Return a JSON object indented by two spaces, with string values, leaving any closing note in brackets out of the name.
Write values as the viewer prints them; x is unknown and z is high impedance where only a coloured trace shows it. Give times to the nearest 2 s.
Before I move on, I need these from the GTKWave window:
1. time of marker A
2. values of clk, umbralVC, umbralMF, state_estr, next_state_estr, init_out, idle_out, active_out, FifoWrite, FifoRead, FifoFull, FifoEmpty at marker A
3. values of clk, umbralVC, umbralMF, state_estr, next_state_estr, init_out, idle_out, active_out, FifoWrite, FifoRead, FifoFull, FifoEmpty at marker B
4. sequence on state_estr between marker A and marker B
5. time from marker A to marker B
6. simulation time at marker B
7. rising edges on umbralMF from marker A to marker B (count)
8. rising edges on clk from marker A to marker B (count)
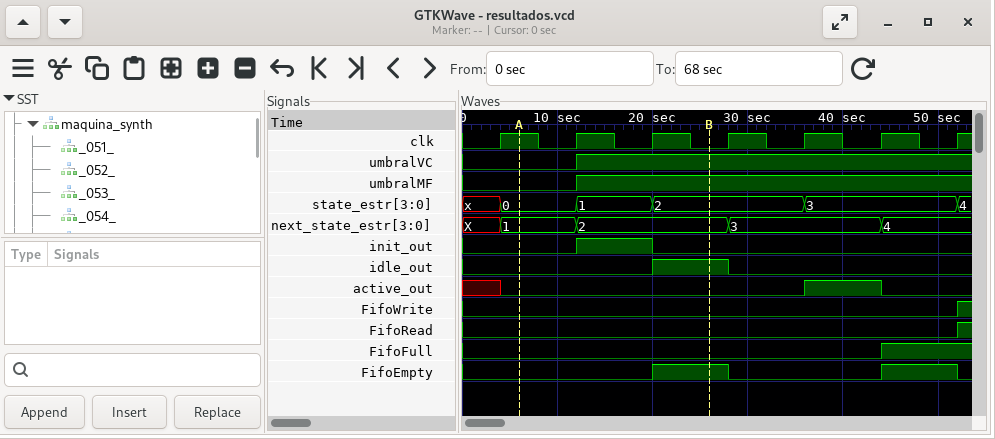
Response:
{
  "time of marker A": "6 s",
  "values of clk, umbralVC, umbralMF, state_estr, next_state_estr, init_out, idle_out, active_out, FifoWrite, FifoRead, FifoFull, FifoEmpty at marker A": "clk=1, umbralVC=0, umbralMF=0, state_estr=0, next_state_estr=1, init_out=0, idle_out=0, active_out=0, FifoWrite=0, FifoRead=0, FifoFull=0, FifoEmpty=0",
  "values of clk, umbralVC, umbralMF, state_estr, next_state_estr, init_out, idle_out, active_out, FifoWrite, FifoRead, FifoFull, FifoEmpty at marker B": "clk=0, umbralVC=1, umbralMF=1, state_estr=2, next_state_estr=2, init_out=0, idle_out=1, active_out=0, FifoWrite=0, FifoRead=0, FifoFull=0, FifoEmpty=1",
  "sequence on state_estr between marker A and marker B": "0, 1, 2",
  "time from marker A to marker B": "20 s",
  "simulation time at marker B": "26 s",
  "rising edges on umbralMF from marker A to marker B": "1",
  "rising edges on clk from marker A to marker B": "2"
}
